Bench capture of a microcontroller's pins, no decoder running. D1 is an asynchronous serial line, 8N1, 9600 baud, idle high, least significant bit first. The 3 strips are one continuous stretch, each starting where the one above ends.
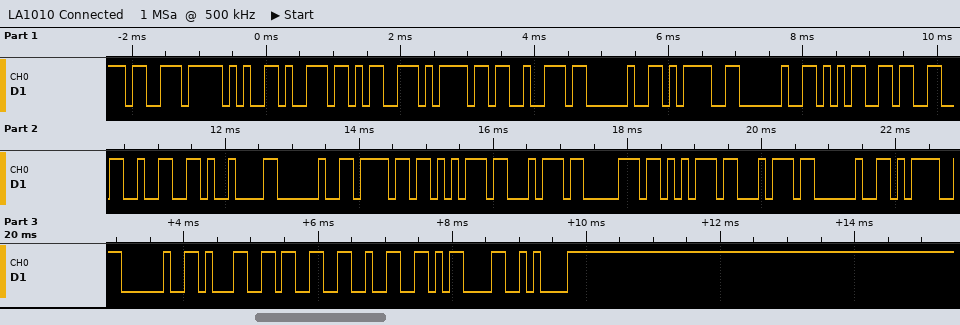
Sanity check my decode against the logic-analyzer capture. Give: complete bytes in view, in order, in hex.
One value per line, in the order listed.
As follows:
73 65 6E 73 6F 72 20 3D 20 35 33 32 09 20 6F 75 74 70 75 74 20 3D 20 31 33 32 0D 0A
